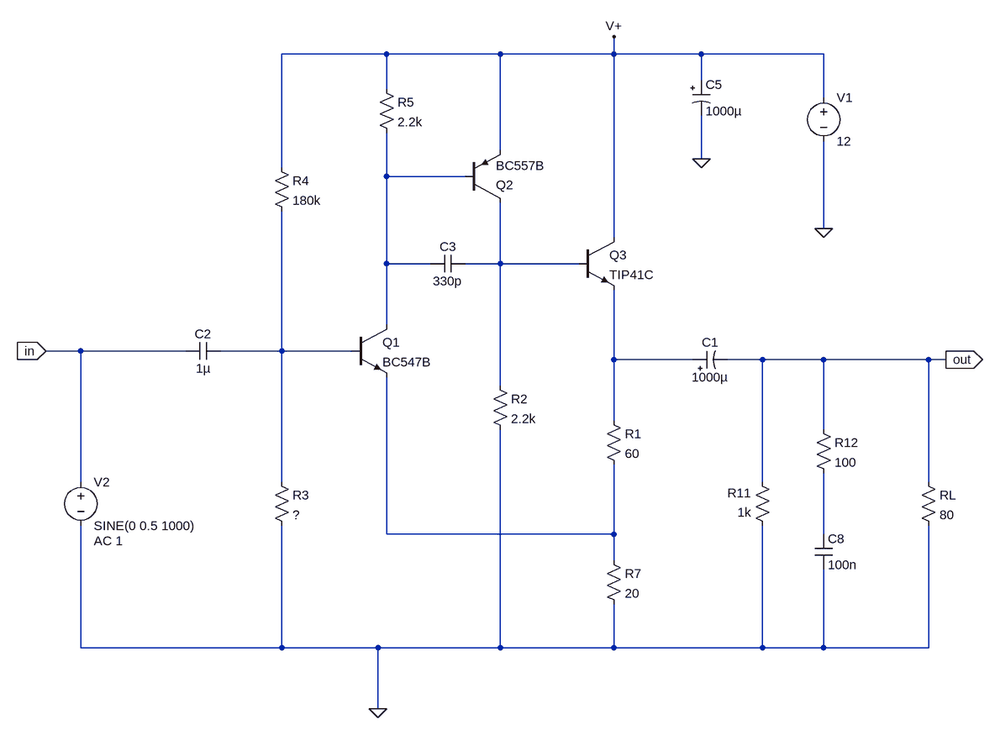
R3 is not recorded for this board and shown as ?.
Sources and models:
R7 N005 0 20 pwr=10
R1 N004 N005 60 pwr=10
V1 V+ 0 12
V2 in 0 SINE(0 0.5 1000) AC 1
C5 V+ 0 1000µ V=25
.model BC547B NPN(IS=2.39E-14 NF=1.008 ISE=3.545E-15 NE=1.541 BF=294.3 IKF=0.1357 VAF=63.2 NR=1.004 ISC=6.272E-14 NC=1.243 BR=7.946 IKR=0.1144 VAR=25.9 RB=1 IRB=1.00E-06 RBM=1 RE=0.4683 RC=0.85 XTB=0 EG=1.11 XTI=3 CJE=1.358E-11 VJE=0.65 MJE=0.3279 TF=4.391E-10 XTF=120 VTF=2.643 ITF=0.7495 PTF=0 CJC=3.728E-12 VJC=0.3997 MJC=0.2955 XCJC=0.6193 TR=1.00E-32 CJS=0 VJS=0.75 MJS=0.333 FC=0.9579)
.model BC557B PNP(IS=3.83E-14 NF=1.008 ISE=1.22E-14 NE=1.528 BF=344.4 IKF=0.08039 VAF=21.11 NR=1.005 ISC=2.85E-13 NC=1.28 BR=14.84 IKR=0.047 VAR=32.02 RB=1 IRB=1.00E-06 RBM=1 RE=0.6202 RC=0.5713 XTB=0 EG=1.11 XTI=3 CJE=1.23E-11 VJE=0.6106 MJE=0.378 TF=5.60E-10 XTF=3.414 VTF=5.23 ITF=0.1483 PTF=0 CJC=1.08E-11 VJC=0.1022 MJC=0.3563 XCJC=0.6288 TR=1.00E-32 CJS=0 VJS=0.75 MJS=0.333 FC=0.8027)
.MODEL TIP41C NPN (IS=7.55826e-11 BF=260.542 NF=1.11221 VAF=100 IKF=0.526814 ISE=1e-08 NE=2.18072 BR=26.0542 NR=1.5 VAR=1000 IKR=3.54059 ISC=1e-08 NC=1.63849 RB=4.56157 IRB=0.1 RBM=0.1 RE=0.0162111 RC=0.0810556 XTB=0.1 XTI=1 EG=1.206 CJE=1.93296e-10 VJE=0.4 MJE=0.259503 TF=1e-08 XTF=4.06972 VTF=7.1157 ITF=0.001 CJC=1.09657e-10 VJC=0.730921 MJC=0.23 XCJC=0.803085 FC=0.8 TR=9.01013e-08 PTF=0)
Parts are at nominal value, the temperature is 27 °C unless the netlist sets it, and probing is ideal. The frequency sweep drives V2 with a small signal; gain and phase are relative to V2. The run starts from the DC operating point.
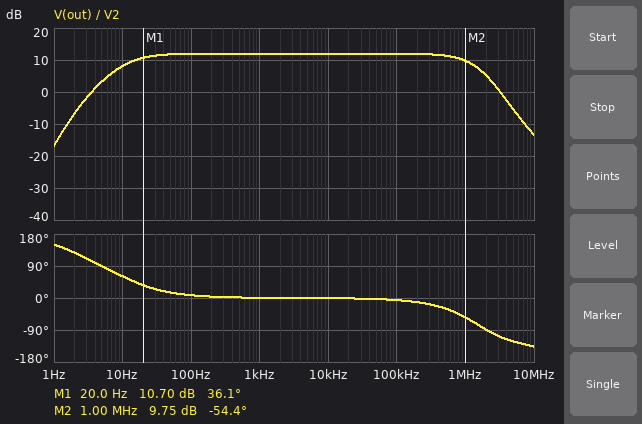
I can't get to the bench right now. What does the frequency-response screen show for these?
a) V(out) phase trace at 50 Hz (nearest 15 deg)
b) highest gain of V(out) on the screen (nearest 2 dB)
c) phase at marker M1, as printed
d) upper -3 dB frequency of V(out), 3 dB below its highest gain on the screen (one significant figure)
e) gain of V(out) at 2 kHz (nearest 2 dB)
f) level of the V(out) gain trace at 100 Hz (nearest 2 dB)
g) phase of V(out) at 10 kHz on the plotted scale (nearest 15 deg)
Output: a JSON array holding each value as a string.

["15 deg", "12 dB", "36.1 deg", "1 MHz", "12 dB", "12 dB", "0 deg"]
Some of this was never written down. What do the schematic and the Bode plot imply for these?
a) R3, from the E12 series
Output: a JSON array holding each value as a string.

["15 kΩ"]
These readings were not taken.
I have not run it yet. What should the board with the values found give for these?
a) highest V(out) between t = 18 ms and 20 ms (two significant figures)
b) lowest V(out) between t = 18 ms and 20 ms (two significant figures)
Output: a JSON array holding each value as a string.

["1.9 V", "-630 mV"]
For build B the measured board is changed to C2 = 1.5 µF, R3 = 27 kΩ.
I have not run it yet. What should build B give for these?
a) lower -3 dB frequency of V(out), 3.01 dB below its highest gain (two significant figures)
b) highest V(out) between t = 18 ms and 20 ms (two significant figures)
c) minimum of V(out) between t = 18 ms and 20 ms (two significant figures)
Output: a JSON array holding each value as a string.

["5.3 Hz", "2.0 V", "-1.8 V"]
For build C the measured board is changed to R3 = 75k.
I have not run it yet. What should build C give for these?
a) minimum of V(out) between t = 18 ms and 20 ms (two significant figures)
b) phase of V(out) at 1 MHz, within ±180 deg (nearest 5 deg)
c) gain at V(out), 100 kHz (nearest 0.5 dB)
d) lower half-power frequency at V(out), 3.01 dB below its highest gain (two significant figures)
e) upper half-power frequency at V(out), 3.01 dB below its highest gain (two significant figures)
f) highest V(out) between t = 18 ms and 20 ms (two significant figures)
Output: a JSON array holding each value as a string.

["-2.6 V", "-30 deg", "3.0 dB", "8.1 Hz", "1.9 MHz", "250 mV"]
